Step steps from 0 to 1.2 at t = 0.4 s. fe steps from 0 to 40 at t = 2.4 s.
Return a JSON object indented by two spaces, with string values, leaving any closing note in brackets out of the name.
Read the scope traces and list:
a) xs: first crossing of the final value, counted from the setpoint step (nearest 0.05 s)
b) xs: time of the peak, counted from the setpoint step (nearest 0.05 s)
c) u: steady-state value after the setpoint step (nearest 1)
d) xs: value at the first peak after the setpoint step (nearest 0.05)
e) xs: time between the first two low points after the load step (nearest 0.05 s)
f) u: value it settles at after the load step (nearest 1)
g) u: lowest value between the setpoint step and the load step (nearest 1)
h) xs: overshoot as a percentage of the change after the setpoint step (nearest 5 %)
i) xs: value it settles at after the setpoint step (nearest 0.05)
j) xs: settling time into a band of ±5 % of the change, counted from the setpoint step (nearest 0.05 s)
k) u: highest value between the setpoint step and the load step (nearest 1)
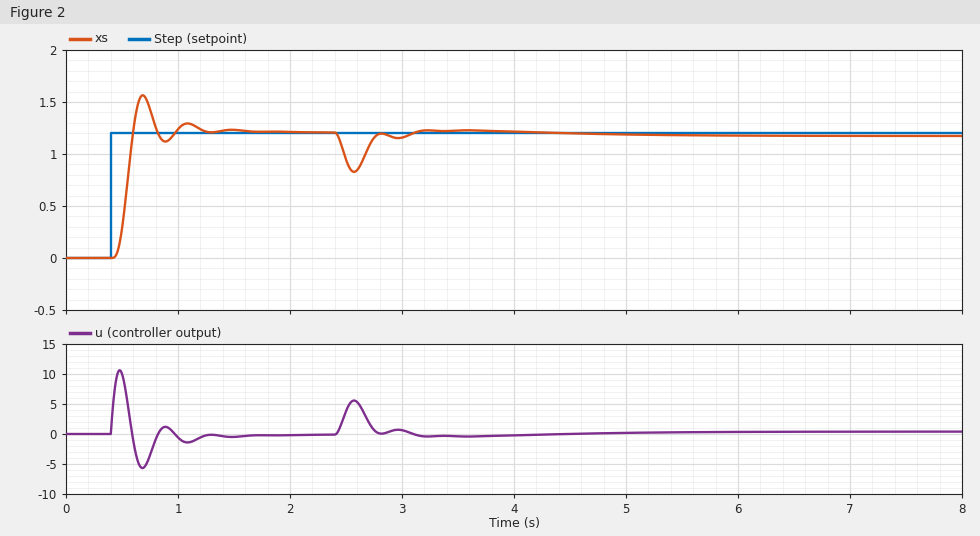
{
  "xs: first crossing of the final value, counted from the setpoint step": "0.20 s",
  "xs: time of the peak, counted from the setpoint step": "0.30 s",
  "u: steady-state value after the setpoint step": "0",
  "xs: value at the first peak after the setpoint step": "1.55",
  "xs: time between the first two low points after the load step": "0.40 s",
  "u: value it settles at after the load step": "0",
  "u: lowest value between the setpoint step and the load step": "-6",
  "xs: overshoot as a percentage of the change after the setpoint step": "30 %",
  "xs: value it settles at after the setpoint step": "1.20",
  "xs: settling time into a band of ±5 % of the change, counted from the setpoint step": "0.75 s",
  "u: highest value between the setpoint step and the load step": "11"
}
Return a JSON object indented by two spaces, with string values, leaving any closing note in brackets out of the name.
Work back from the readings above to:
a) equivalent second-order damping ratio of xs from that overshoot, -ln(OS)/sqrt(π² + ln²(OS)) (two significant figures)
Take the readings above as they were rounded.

{
  "equivalent second-order damping ratio of xs from that overshoot, -ln(OS)/sqrt(π² + ln²(OS))": "0.36"
}
